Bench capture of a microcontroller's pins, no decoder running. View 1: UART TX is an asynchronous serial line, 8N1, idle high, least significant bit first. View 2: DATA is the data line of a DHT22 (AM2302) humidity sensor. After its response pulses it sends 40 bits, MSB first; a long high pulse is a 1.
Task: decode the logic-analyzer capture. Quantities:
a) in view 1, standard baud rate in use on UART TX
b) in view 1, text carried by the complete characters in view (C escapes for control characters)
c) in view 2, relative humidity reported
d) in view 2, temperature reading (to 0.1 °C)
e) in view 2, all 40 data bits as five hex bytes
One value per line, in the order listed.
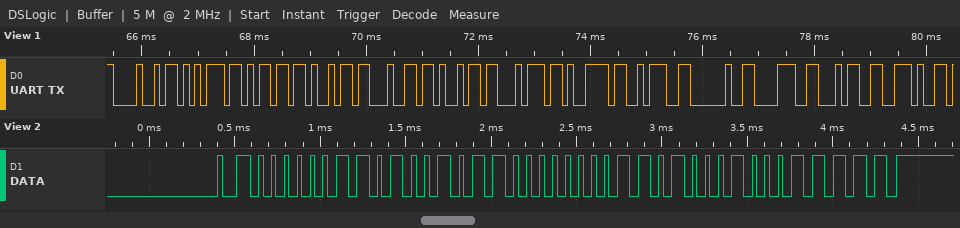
9600 baud
"Humidity: 84."
84.3 %
20.9 °C
03 4B 00 D1 1F
